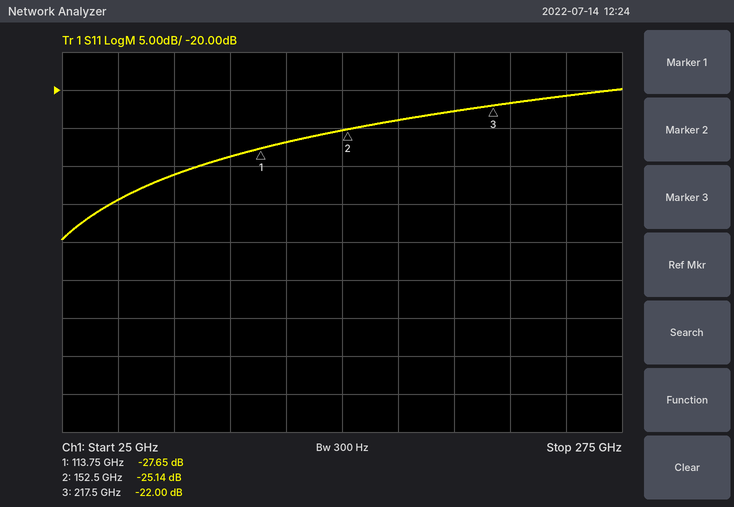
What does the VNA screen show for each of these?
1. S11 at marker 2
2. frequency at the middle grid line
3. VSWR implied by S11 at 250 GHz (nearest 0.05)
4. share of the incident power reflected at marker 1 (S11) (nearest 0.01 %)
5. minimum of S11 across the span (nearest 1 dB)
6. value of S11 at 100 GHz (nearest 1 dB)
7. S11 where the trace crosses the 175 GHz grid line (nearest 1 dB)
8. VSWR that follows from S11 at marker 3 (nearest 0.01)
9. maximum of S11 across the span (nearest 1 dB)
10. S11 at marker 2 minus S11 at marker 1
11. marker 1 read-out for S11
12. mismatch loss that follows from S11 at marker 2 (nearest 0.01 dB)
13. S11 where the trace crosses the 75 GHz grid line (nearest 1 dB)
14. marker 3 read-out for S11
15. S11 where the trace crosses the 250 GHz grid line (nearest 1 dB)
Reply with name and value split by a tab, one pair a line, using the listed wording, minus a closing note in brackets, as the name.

S11 at marker 2	-25.14 dB
frequency at the middle grid line	150 GHz
VSWR implied by S11 at 250 GHz	1.20
share of the incident power reflected at marker 1 (S11)	0.17 %
minimum of S11 across the span	-40 dB
value of S11 at 100 GHz	-29 dB
S11 where the trace crosses the 175 GHz grid line	-24 dB
VSWR that follows from S11 at marker 3	1.17
maximum of S11 across the span	-20 dB
S11 at marker 2 minus S11 at marker 1	2.51 dB
marker 1 read-out for S11	-27.65 dB
mismatch loss that follows from S11 at marker 2	0.01 dB
S11 where the trace crosses the 75 GHz grid line	-31 dB
marker 3 read-out for S11	-22.00 dB
S11 where the trace crosses the 250 GHz grid line	-21 dB
